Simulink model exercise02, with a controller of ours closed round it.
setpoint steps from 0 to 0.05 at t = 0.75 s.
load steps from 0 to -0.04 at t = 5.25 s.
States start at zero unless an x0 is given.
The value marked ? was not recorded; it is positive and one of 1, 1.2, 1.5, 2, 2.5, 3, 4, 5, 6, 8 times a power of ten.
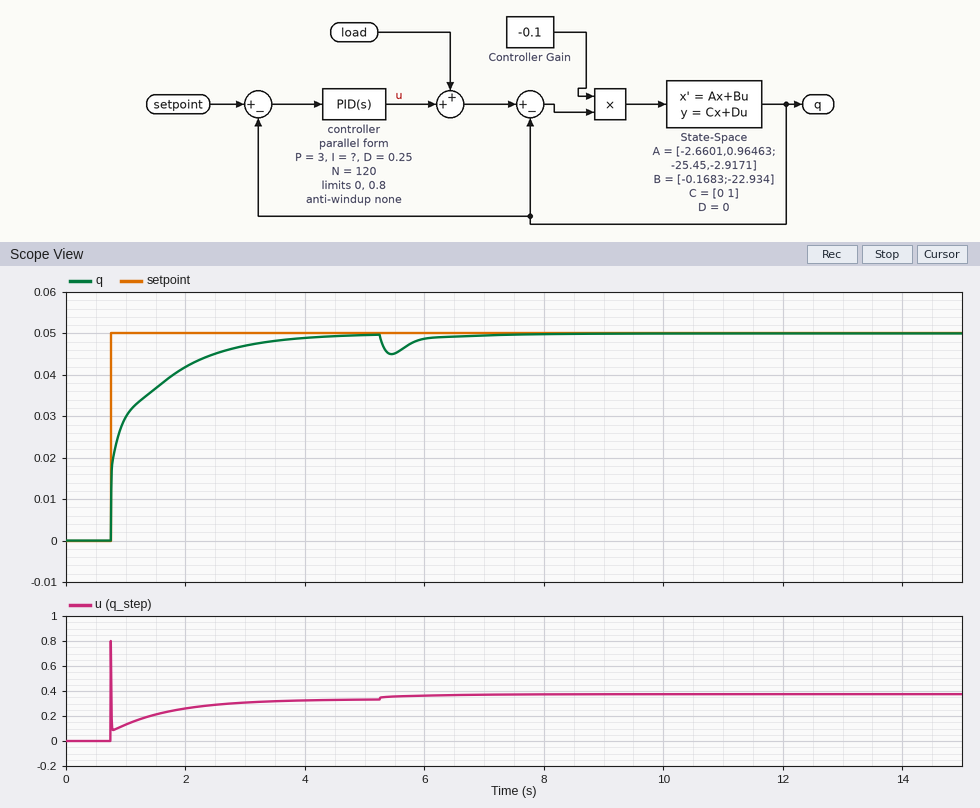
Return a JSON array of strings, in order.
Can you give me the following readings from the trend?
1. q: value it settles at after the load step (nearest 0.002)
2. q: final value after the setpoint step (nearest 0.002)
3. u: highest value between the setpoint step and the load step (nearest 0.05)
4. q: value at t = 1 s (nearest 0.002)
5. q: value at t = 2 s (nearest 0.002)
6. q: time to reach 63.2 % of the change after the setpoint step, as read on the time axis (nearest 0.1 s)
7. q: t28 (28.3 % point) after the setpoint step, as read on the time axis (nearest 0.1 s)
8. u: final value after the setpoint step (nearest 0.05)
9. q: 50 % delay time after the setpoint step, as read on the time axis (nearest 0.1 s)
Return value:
["0.050", "0.050", "0.80", "0.030", "0.042", "1.1 s", "0.8 s", "0.35", "0.9 s"]
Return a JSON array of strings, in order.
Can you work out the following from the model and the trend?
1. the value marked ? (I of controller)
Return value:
["12"]
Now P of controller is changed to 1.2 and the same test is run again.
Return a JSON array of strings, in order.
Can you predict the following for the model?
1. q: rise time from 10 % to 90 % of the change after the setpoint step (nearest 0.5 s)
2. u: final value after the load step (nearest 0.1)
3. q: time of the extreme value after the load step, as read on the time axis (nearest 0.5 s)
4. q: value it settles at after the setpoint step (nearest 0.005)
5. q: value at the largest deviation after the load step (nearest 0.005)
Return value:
["1.5 s", "0.4", "5.5 s", "0.050", "0.045"]
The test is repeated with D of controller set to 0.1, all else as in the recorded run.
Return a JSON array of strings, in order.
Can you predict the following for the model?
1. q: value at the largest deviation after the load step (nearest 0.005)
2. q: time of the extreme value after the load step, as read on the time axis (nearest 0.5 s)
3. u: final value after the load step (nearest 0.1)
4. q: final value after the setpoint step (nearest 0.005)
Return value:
["0.045", "5.5 s", "0.4", "0.050"]
